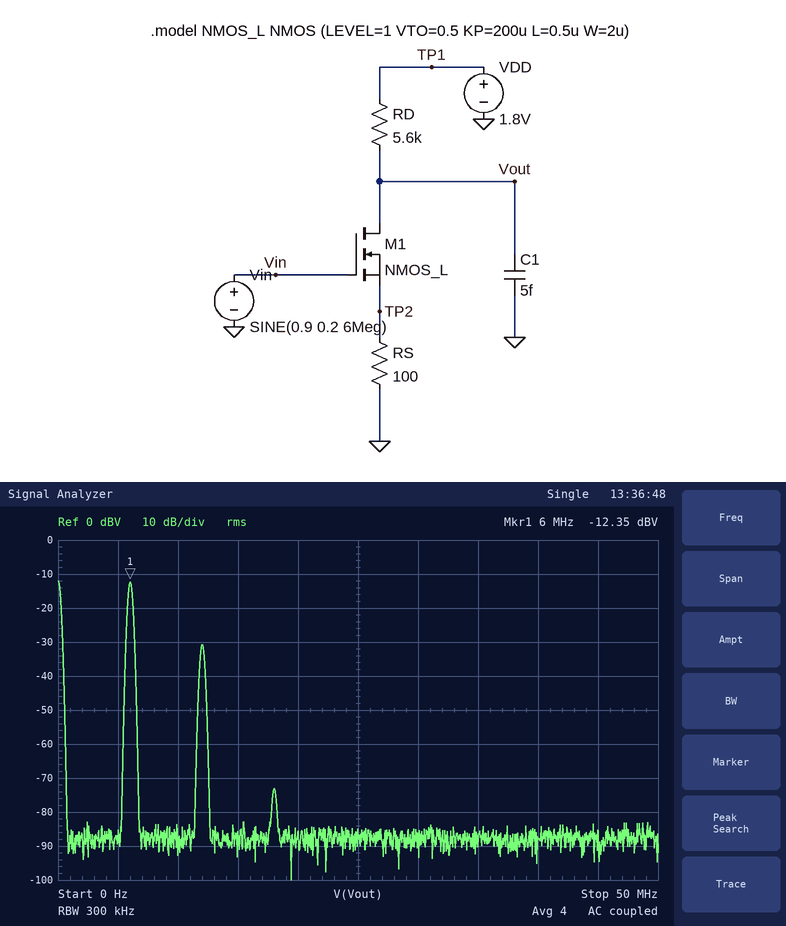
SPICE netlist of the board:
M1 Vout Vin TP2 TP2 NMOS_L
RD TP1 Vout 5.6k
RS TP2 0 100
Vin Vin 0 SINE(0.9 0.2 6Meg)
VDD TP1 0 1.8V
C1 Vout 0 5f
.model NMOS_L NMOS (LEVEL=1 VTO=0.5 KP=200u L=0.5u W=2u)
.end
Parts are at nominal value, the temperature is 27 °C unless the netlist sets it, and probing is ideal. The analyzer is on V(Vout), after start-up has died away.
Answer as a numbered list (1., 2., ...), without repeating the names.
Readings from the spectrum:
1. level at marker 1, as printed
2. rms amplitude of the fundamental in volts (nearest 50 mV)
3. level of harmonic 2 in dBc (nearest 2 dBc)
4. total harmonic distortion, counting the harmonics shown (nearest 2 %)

1. -12.35 dBV
2. 250 mV
3. -18 dBc
4. 12 %
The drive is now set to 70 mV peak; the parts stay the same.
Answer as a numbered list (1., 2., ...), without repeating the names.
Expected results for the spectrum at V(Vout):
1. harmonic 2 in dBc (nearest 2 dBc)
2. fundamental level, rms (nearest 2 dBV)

1. -28 dBc
2. -22 dBV
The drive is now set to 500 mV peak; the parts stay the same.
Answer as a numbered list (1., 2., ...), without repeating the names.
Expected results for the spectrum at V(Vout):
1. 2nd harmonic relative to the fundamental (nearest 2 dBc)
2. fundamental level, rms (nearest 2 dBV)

1. -14 dBc
2. -6 dBV
